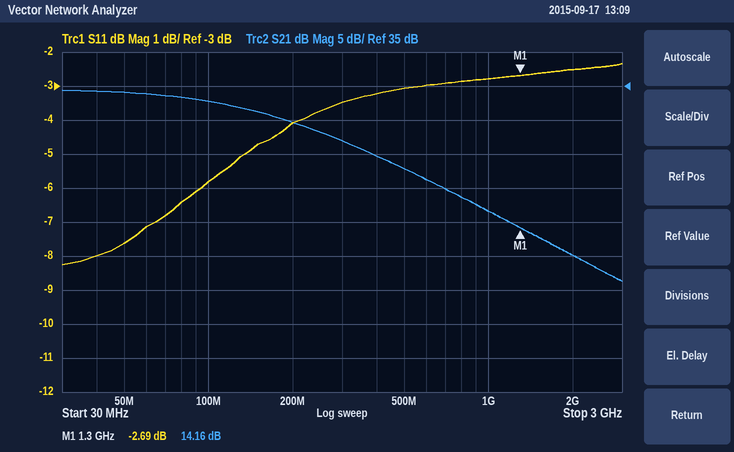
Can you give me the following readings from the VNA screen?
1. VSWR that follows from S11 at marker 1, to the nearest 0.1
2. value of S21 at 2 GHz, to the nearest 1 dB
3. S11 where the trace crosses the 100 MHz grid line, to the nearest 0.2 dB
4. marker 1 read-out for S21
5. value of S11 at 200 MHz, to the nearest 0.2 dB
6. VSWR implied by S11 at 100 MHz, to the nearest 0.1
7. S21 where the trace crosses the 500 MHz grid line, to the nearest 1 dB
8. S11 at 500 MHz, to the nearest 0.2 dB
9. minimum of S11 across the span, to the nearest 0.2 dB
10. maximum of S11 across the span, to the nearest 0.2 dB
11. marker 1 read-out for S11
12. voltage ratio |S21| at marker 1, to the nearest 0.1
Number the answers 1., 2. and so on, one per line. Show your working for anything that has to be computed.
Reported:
1. (1 + 0.7337)/(1 − 0.7337) ≈ 6.5
2. 10 dB
3. -5.8 dB
4. 14.16 dB
5. -4.0 dB
6. |Γ| = 10^(-5.8/20) = 0.5129; VSWR = (1 + 0.5129)/(1 − 0.5129) ≈ 3.1
7. 23 dB
8. -3.0 dB
9. -8.2 dB
10. -2.4 dB
11. -2.69 dB
12. 10^(14.16/20) ≈ 5.1
